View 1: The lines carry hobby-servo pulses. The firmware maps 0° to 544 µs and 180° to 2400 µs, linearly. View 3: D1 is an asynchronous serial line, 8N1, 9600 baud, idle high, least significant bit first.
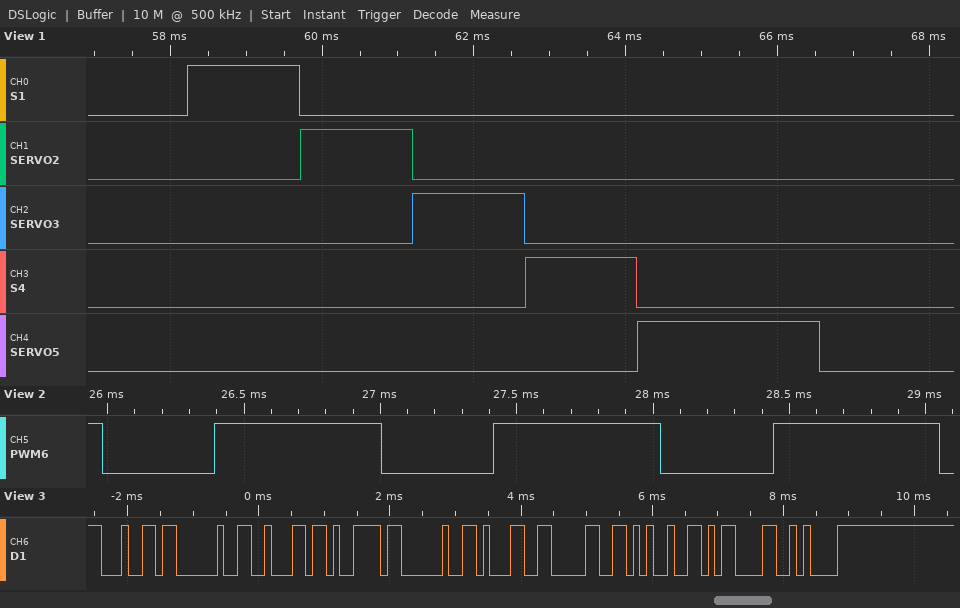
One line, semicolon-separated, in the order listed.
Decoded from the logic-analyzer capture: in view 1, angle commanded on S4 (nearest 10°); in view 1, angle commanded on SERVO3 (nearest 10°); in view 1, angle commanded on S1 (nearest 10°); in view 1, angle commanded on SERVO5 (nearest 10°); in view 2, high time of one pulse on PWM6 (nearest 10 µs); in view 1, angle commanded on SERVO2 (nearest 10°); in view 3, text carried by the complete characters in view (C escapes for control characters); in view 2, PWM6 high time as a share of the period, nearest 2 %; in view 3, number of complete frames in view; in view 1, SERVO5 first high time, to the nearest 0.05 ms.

90°; 90°; 90°; 180°; 610 µs; 90°; "d by 10%\r\n"; 60 %; 10; 2.40 ms
